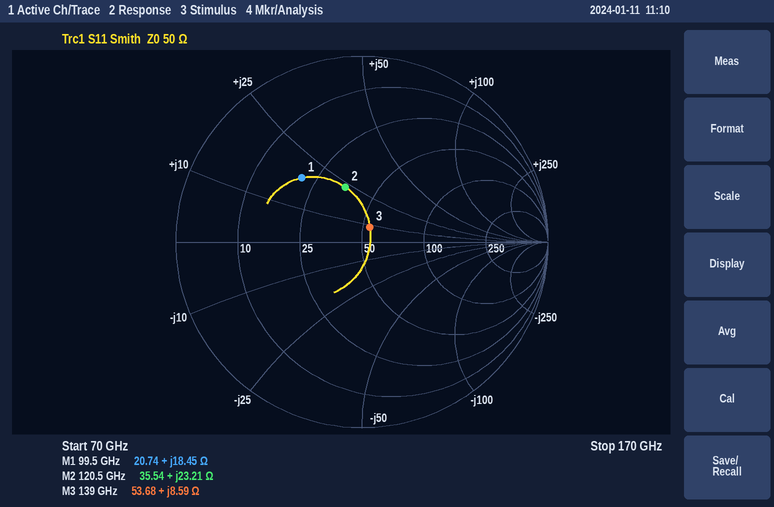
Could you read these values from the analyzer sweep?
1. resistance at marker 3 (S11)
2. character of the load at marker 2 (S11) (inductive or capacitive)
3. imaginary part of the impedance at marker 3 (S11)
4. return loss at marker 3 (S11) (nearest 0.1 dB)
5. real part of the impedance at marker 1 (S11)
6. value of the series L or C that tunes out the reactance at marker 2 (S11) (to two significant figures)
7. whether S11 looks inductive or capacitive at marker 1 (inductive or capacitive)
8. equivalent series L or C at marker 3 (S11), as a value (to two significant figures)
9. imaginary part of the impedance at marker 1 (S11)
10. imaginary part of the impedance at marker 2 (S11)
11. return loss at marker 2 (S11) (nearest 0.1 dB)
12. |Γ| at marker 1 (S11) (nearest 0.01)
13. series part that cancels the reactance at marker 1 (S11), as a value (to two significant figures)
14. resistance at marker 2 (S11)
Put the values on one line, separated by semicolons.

53.68 Ω; inductive; +8.59 Ω; 20.9 dB; 20.74 Ω; 57 fF; inductive; 9.8 pH; +18.45 Ω; +23.21 Ω; 10.2 dB; 0.47; 87 fF; 35.54 Ω
